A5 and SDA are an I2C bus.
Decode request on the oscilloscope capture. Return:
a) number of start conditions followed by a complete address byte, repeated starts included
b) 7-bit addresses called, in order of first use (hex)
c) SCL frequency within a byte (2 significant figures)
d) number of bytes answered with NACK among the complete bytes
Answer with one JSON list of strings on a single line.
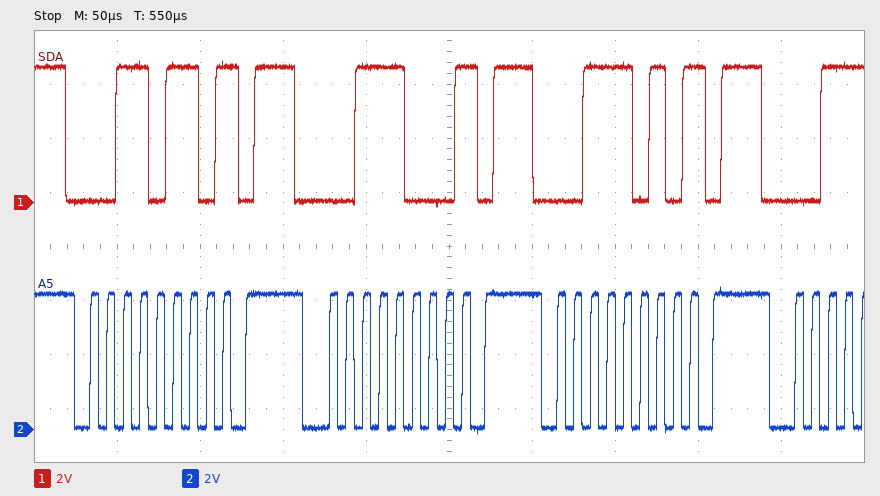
["3", "0x1B 0x1C 0x1D", "100 kHz", "3"]
